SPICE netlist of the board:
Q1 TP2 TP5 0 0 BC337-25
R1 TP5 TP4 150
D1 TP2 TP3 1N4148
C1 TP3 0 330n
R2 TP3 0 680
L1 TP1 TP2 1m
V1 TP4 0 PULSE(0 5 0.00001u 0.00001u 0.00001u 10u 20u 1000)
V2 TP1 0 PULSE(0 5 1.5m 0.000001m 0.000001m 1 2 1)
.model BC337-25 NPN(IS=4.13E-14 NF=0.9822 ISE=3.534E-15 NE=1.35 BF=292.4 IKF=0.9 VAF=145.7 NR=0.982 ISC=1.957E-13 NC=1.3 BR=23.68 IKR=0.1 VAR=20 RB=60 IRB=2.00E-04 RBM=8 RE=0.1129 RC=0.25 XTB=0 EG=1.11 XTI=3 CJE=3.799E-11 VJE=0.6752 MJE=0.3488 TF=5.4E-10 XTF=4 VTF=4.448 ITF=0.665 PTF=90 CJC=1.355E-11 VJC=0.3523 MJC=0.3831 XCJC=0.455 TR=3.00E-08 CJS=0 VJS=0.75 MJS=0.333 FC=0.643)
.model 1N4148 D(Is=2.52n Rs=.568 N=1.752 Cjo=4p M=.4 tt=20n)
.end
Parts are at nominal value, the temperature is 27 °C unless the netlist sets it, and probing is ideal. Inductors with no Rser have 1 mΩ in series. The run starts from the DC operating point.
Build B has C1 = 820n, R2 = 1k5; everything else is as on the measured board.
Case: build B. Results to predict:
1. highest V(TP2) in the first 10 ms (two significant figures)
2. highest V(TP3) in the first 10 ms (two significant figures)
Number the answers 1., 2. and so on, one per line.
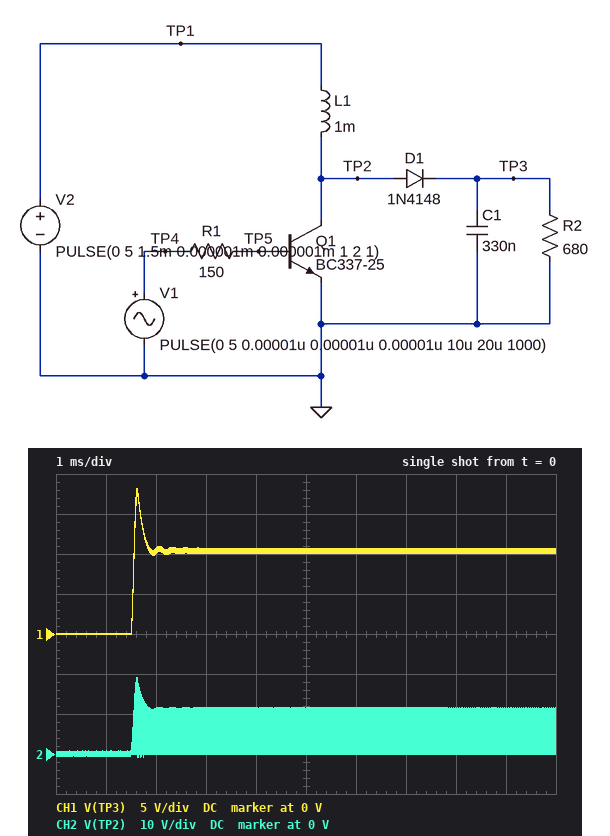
1. 20 V
2. 19 V
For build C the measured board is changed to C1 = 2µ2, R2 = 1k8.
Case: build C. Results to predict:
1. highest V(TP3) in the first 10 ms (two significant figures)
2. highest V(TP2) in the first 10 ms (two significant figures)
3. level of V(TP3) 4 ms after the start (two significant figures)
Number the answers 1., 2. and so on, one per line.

1. 19 V
2. 20 V
3. 16 V
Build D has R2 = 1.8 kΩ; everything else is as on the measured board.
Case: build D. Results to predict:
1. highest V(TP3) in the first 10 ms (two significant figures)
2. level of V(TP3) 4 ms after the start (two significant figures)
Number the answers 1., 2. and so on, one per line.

1. 19 V
2. 14 V
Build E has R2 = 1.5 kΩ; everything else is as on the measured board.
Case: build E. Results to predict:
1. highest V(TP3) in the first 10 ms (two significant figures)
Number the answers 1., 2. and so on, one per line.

1. 19 V
